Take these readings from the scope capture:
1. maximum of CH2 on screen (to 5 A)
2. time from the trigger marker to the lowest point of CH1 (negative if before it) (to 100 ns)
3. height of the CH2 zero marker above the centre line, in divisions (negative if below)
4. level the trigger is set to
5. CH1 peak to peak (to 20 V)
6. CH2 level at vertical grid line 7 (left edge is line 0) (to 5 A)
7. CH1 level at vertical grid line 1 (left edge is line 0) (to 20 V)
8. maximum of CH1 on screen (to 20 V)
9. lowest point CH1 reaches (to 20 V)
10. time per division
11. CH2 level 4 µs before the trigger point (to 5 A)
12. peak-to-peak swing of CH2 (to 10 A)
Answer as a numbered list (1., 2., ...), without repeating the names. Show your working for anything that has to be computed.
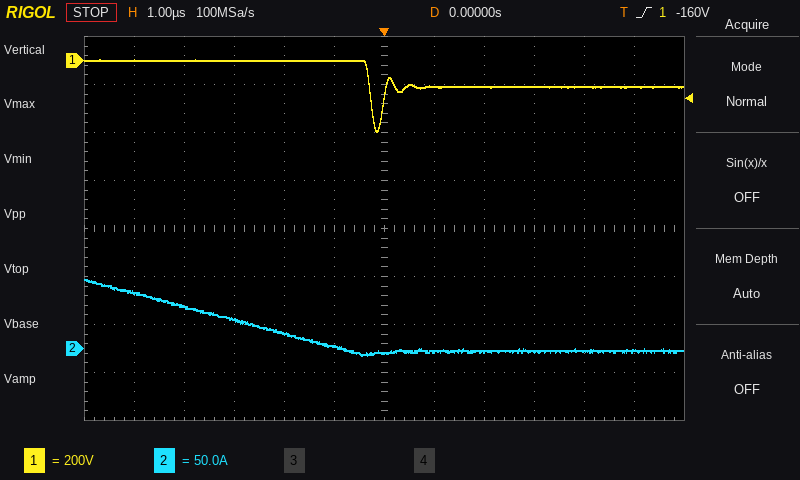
1. 70 A
2. -100 ns
3. -2.5 div
4. -160 V
5. 0 V − (-300 V) = 300 V
6. -5 A
7. 0 V
8. 0 V
9. -300 V
10. 1 µs
11. 45 A
12. 80 A
